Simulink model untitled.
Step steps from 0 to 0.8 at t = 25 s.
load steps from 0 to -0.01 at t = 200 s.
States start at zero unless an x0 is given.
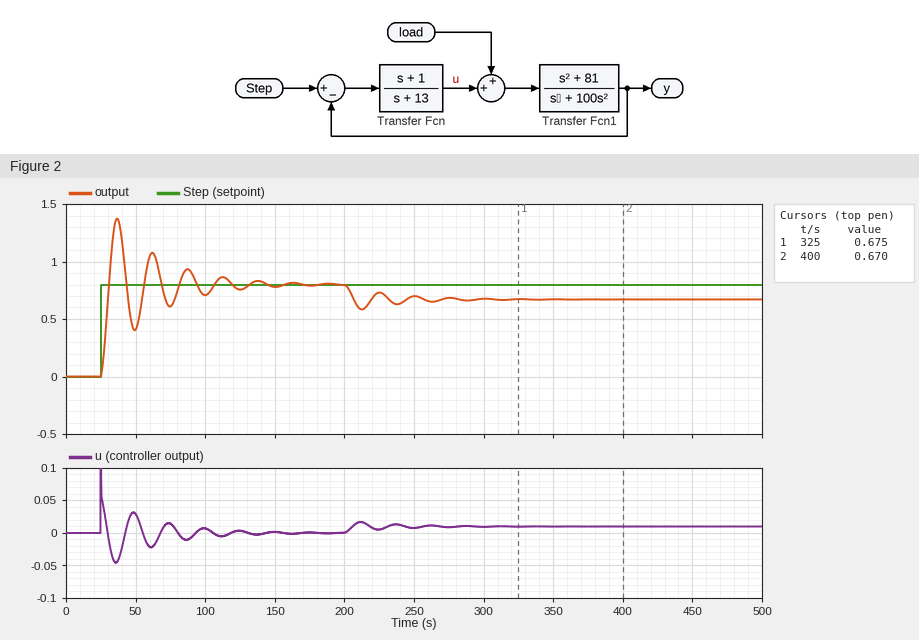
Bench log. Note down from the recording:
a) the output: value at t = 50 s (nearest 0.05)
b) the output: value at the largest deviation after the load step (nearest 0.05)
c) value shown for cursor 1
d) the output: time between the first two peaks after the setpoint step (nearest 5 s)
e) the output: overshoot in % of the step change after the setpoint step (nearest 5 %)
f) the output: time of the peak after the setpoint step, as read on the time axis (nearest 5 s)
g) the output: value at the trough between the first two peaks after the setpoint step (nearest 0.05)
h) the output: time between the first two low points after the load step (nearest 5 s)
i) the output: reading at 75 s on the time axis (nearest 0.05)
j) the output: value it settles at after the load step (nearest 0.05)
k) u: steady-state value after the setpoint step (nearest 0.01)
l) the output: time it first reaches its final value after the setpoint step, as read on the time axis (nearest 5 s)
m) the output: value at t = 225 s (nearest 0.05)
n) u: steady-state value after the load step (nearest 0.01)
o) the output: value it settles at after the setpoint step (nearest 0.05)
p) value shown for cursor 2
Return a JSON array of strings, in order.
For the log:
["0.40", "0.60", "0.675", "25 s", "70 %", "35 s", "0.40", "25 s", "0.60", "0.65", "0.00", "30 s", "0.75", "0.01", "0.80", "0.670"]
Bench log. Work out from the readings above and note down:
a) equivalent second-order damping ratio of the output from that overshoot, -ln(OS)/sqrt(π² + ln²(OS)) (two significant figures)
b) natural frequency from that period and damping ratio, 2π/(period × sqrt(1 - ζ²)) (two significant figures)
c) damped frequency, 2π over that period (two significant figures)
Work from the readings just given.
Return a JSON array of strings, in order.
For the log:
["0.11", "0.25 rad/s", "0.25 rad/s"]
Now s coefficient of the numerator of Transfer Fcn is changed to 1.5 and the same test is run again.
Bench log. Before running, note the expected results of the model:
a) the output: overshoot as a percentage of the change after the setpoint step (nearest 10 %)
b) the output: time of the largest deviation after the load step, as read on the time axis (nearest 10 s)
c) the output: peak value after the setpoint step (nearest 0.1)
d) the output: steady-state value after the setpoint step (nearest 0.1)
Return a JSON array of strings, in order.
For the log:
["60 %", "210 s", "1.3", "0.8"]
